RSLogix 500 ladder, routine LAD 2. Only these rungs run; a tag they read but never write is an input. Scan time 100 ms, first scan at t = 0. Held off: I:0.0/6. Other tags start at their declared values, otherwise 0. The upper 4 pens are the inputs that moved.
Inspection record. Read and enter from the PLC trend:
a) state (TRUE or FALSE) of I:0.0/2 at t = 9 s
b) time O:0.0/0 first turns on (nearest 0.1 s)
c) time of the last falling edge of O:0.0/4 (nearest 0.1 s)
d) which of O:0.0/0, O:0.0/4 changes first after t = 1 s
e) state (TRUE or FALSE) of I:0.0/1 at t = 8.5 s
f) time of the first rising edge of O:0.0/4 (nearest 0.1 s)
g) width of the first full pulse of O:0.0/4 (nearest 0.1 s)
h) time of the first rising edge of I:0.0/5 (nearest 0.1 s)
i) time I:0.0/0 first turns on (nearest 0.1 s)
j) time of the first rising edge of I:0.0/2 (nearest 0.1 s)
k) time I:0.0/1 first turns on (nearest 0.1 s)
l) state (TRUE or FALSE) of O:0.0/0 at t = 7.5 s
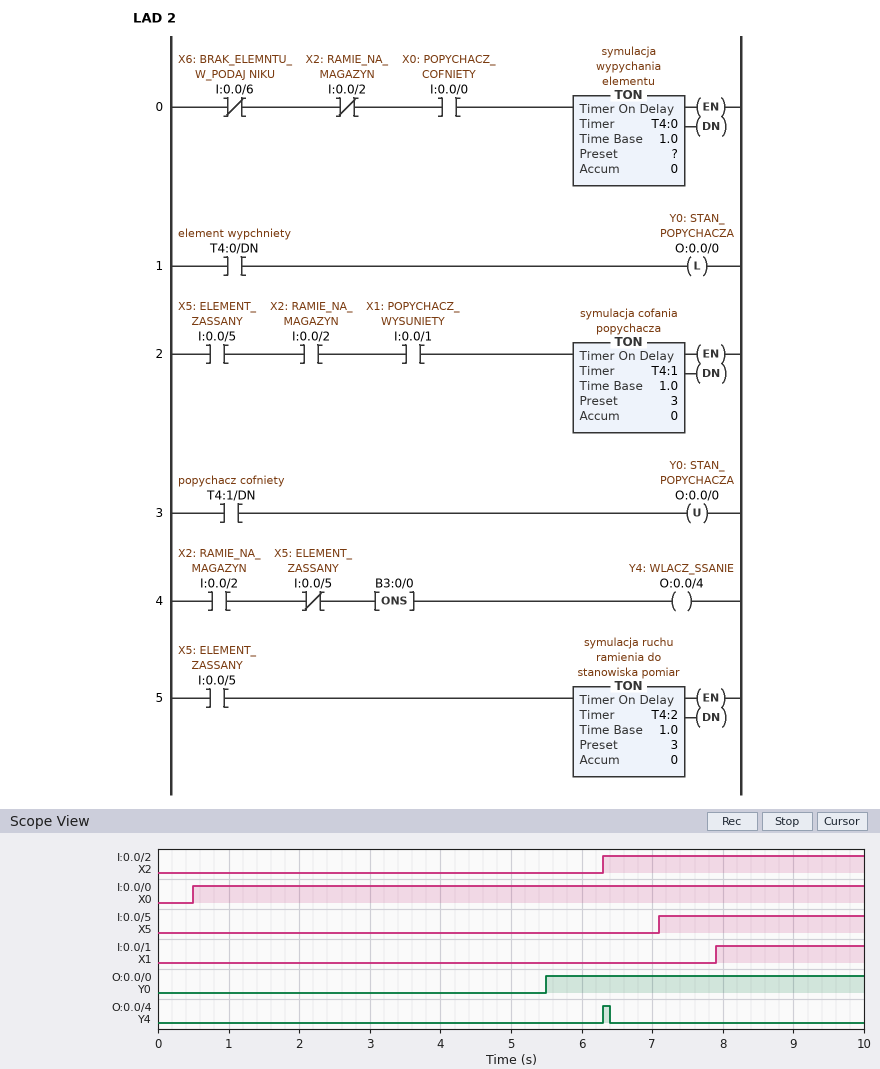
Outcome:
TRUE
5.5 s
6.4 s
O:0.0/0
TRUE
6.3 s
0.1 s
7.1 s
0.5 s
6.3 s
7.9 s
TRUE
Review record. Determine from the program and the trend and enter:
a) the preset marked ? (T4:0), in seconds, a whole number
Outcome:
5 s
